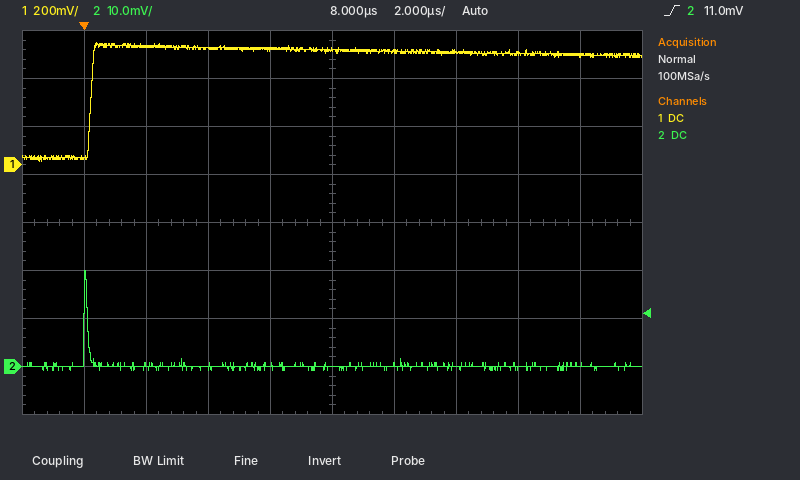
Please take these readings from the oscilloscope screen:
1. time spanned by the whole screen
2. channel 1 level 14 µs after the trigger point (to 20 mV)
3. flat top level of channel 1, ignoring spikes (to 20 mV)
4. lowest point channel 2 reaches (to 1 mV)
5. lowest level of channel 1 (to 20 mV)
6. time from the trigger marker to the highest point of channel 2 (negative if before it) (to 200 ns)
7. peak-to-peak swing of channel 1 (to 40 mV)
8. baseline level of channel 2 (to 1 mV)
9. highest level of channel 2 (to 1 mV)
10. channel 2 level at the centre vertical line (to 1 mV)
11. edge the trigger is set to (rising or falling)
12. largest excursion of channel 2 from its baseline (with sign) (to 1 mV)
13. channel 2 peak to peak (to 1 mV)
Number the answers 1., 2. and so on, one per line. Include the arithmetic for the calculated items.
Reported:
1. 20 µs
2. 460 mV
3. 480 mV
4. -1 mV
5. 20 mV
6. 0.0 µs
7. 480 mV
8. 0 mV
9. 20 mV
10. 0 mV
11. rising
12. 20 mV − (0 mV) = +20 mV
13. 20 mV − (-1 mV) = 21 mV
